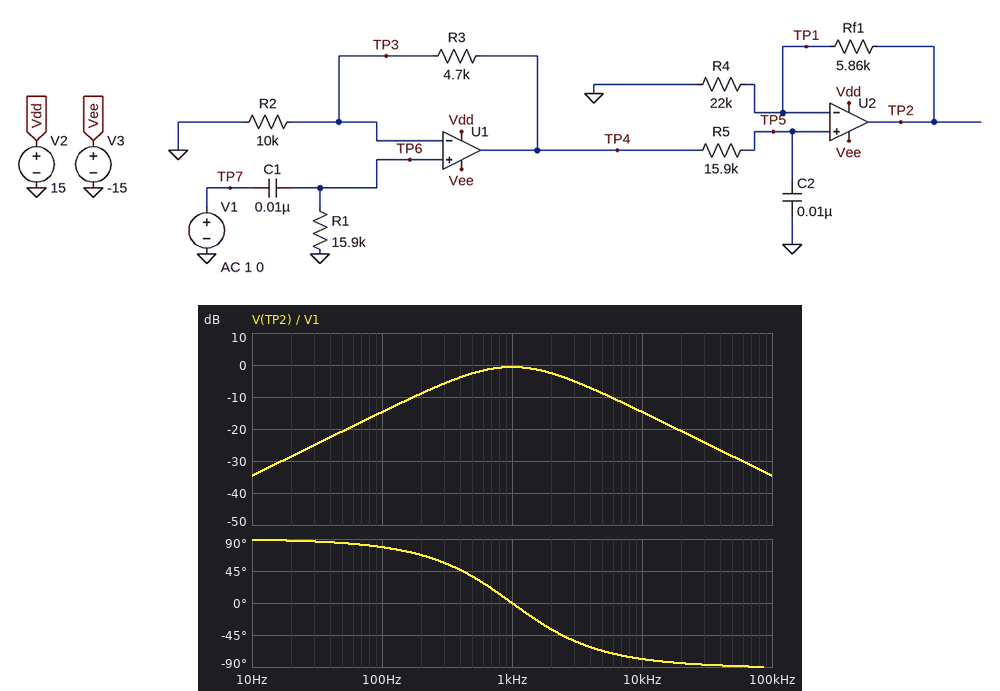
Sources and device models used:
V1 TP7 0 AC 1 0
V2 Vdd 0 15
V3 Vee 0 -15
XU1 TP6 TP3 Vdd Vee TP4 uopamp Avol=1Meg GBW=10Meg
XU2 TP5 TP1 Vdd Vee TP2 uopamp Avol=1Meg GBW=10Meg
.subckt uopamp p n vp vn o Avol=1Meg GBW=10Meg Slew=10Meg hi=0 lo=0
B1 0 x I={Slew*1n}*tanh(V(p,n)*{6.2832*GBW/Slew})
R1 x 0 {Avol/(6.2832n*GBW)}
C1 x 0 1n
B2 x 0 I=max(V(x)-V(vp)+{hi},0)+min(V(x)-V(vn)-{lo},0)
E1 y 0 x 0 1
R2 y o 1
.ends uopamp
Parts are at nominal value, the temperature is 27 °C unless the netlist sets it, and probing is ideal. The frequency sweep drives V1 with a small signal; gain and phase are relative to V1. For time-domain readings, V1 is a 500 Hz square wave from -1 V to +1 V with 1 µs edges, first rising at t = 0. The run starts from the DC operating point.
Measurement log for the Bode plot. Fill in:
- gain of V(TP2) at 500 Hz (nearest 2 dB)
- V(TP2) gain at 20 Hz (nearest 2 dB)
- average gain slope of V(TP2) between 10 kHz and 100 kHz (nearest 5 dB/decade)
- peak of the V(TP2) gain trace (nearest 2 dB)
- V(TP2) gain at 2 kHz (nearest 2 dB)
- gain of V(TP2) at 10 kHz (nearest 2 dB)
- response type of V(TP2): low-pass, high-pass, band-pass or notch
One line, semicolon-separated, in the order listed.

-2 dB; -28 dB; -20 dB/decade; 0 dB; -2 dB; -14 dB; band-pass
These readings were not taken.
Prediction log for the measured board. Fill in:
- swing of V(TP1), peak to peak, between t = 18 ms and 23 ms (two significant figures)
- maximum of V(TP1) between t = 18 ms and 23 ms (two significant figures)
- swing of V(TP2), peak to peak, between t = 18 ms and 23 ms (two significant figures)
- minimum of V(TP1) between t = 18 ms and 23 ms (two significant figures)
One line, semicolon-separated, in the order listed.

2.1 V; 1.1 V; 2.7 V; -1.1 V
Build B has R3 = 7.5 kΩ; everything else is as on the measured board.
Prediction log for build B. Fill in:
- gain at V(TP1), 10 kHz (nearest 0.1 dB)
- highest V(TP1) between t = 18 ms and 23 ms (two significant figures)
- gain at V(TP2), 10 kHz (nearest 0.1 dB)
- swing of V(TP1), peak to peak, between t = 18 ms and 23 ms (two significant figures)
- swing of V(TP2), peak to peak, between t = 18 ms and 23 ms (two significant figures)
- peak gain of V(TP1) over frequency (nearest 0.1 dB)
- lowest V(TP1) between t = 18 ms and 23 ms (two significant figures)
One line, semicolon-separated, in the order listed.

-15.2 dB; 1.3 V; -13.2 dB; 2.5 V; 3.2 V; -1.2 dB; -1.3 V
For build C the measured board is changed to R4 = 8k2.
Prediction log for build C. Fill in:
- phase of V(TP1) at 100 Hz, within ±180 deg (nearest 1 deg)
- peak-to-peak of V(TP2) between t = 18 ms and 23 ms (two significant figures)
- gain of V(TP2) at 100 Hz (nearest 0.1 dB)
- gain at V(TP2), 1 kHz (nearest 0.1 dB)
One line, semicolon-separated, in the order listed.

79 deg; 3.7 V; -12.1 dB; 2.0 dB
